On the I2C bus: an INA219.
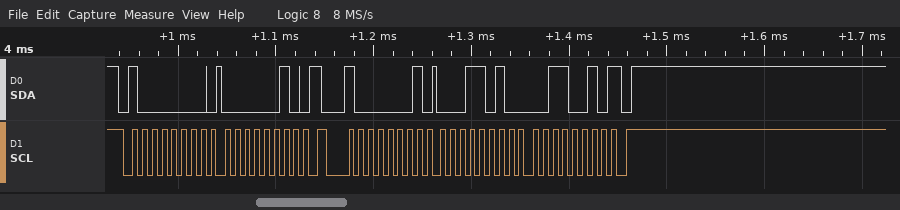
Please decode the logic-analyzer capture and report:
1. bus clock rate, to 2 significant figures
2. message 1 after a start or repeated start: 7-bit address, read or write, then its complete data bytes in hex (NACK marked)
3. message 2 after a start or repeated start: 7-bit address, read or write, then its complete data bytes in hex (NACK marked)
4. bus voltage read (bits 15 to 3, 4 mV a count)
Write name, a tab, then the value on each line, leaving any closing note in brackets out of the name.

bus clock rate, to 2 significant figures	100 kHz
message 1 after a start or repeated start: 7-bit address, read or write, then its complete data bytes in hex	0x40 write: 02
message 2 after a start or repeated start: 7-bit address, read or write, then its complete data bytes in hex	0x40 read: 1A 32 NACK
bus voltage read	3.352 V
